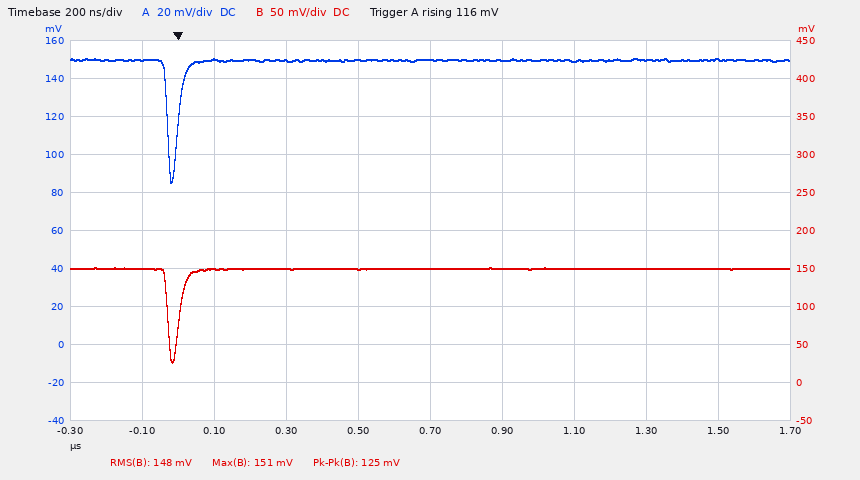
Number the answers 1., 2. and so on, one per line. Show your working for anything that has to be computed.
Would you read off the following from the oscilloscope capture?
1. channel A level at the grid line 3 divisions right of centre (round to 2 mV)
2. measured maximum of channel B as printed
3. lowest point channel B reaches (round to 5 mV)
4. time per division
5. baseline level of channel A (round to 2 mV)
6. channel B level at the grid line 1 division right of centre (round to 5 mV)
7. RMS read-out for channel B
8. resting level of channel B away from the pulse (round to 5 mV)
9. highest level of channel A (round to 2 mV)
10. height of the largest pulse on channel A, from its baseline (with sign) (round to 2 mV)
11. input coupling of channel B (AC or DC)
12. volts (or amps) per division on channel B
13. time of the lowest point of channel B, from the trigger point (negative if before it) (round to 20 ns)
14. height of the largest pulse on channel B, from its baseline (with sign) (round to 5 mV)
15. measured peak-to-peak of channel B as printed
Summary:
1. 150 mV
2. 151 mV
3. 25 mV
4. 200 ns
5. 150 mV
6. 150 mV
7. 148 mV
8. 150 mV
9. 150 mV
10. -64 mV
11. DC
12. 50 mV
13. -20 ns
14. 25 mV − (150 mV) = -125 mV
15. 125 mV
